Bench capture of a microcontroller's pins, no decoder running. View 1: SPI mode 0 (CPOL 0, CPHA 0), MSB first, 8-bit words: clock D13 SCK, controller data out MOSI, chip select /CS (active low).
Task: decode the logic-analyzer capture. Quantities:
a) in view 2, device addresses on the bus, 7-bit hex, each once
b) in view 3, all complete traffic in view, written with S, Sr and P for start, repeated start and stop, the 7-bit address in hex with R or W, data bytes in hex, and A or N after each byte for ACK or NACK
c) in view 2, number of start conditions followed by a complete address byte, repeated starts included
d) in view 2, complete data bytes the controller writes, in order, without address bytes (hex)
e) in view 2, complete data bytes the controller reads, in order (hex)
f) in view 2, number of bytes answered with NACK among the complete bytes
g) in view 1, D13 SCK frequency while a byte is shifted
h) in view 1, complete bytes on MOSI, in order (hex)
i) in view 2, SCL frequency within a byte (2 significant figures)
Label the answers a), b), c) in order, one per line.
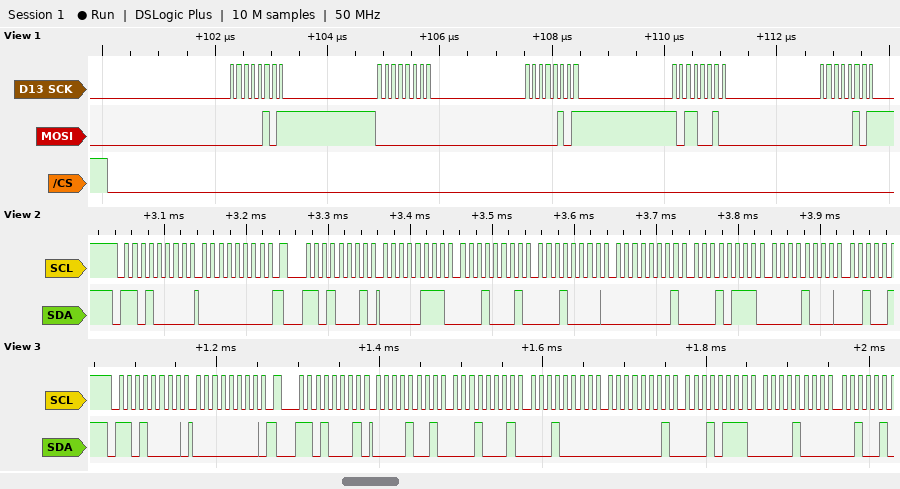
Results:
a) 0x68
b) S 68W A 00 A Sr 68R A 09 A 11 A 10 A 01 A 17 A 08 A
c) 2
d) 00
e) 07 11 10 01 17 08
f) 0
g) 8 MHz
h) 0x05 0x00 0x05 0xB2 0x05
i) 100 kHz
